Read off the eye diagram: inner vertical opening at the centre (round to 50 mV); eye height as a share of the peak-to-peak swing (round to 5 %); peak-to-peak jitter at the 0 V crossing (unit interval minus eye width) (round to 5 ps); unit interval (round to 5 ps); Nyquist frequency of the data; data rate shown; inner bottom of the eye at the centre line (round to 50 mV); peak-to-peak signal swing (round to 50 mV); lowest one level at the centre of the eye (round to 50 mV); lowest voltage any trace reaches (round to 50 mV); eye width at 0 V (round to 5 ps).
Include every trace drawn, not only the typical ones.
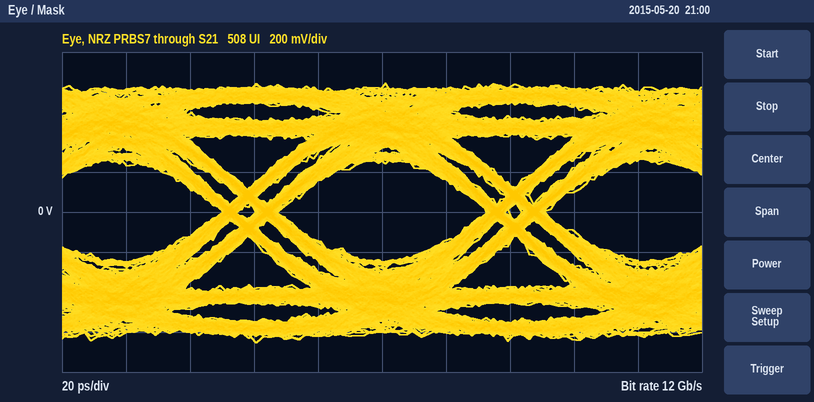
500 mV
40 %
20 ps
85 ps
6 GHz
12 Gb/s
-250 mV
1.30 V
250 mV
-650 mV
65 ps
